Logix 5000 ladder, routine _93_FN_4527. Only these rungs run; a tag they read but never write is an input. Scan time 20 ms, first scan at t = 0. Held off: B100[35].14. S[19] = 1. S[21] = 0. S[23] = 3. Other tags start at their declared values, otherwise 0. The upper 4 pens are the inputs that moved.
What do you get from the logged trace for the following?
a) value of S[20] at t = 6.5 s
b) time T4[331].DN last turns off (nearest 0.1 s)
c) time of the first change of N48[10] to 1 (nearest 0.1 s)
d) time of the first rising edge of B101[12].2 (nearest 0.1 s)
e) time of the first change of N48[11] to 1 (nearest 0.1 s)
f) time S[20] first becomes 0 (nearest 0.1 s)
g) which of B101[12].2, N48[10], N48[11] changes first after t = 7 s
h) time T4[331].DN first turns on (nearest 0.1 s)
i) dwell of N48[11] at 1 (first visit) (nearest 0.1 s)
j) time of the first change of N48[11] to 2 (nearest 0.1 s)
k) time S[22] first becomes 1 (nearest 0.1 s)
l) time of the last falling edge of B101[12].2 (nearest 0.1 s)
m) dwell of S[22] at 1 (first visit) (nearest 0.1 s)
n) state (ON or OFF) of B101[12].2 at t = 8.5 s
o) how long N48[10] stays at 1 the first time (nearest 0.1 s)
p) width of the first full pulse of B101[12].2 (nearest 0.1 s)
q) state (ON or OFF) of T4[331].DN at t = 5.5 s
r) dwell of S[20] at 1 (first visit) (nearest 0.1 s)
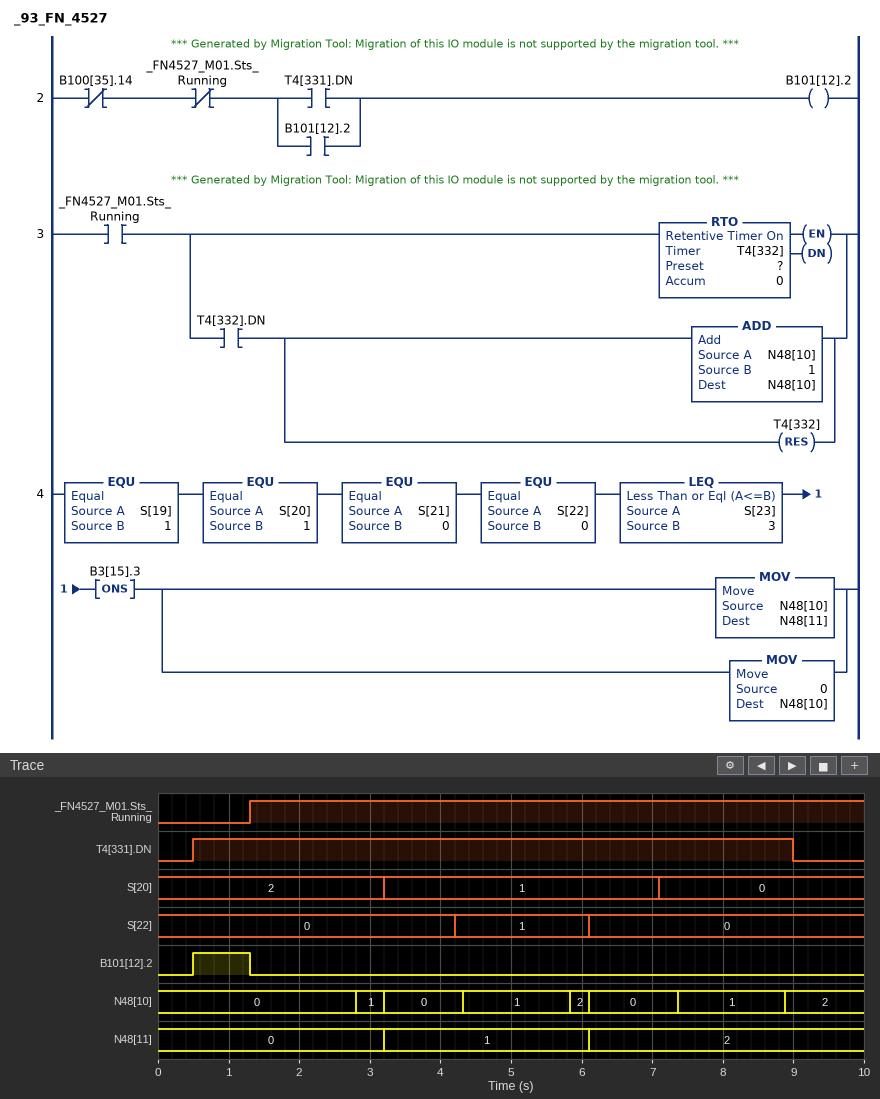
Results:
1
9.0 s
2.8 s
0.5 s
3.2 s
7.1 s
N48[10]
0.5 s
2.9 s
6.1 s
4.2 s
1.3 s
1.9 s
OFF
0.4 s
0.8 s
ON
3.9 s
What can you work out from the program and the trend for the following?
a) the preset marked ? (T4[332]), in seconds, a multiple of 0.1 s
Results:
1.5 s
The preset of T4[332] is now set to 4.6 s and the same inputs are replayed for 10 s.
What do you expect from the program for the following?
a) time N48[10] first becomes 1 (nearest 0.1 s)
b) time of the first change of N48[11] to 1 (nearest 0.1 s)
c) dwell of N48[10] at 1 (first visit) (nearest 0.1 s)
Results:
5.9 s
6.1 s
0.2 s
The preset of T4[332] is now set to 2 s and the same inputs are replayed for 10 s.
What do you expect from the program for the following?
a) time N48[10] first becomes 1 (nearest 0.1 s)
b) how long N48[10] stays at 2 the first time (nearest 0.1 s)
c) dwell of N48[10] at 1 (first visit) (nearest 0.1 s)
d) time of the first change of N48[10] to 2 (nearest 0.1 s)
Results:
3.3 s
0.8 s
2.0 s
5.3 s
